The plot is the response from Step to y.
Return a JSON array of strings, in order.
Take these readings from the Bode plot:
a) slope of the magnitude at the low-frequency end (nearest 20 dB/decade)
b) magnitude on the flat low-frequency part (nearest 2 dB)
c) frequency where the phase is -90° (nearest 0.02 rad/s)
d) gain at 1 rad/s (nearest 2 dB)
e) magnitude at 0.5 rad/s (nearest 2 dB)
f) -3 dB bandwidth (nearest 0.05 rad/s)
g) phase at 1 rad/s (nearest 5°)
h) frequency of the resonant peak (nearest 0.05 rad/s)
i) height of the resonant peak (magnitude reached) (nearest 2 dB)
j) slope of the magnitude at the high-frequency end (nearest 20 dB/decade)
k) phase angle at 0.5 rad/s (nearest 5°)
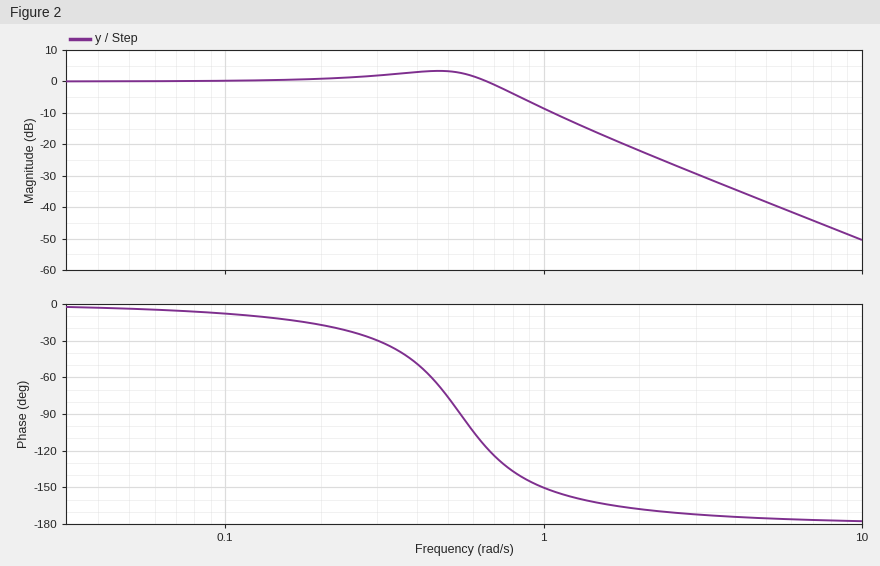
["0 dB/decade", "0 dB", "0.54 rad/s", "-8 dB", "4 dB", "0.75 rad/s", "-150°", "0.45 rad/s", "4 dB", "-40 dB/decade", "-75°"]
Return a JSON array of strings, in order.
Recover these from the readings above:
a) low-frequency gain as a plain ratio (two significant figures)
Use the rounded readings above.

["1.0"]
